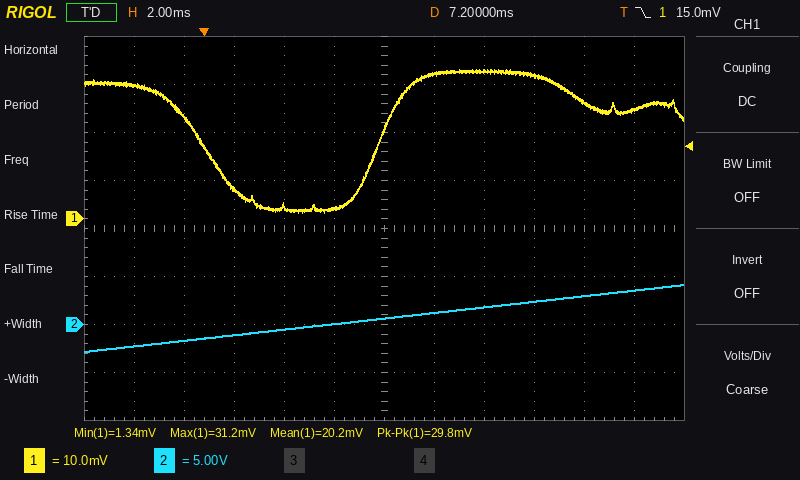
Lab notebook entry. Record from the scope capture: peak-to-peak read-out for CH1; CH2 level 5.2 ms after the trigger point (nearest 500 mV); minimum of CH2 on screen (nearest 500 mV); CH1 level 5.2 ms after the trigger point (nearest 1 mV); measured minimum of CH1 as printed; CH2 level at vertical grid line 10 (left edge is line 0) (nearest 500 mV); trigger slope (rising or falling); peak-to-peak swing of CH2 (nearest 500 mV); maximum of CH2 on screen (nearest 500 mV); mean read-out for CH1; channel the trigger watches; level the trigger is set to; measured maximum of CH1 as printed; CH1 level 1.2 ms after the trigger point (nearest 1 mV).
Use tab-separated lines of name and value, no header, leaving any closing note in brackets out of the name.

peak-to-peak read-out for CH1	29.8 mV
CH2 level 5.2 ms after the trigger point	0.0 V
minimum of CH2 on screen	-3.0 V
CH1 level 5.2 ms after the trigger point	2 mV
measured minimum of CH1 as printed	1.34 mV
CH2 level at vertical grid line 10 (left edge is line 0)	3.0 V
trigger slope	falling
peak-to-peak swing of CH2	7.0 V
maximum of CH2 on screen	4.0 V
mean read-out for CH1	20.2 mV
channel the trigger watches	CH1
level the trigger is set to	15.0 mV
measured maximum of CH1 as printed	31.2 mV
CH1 level 1.2 ms after the trigger point	6 mV
